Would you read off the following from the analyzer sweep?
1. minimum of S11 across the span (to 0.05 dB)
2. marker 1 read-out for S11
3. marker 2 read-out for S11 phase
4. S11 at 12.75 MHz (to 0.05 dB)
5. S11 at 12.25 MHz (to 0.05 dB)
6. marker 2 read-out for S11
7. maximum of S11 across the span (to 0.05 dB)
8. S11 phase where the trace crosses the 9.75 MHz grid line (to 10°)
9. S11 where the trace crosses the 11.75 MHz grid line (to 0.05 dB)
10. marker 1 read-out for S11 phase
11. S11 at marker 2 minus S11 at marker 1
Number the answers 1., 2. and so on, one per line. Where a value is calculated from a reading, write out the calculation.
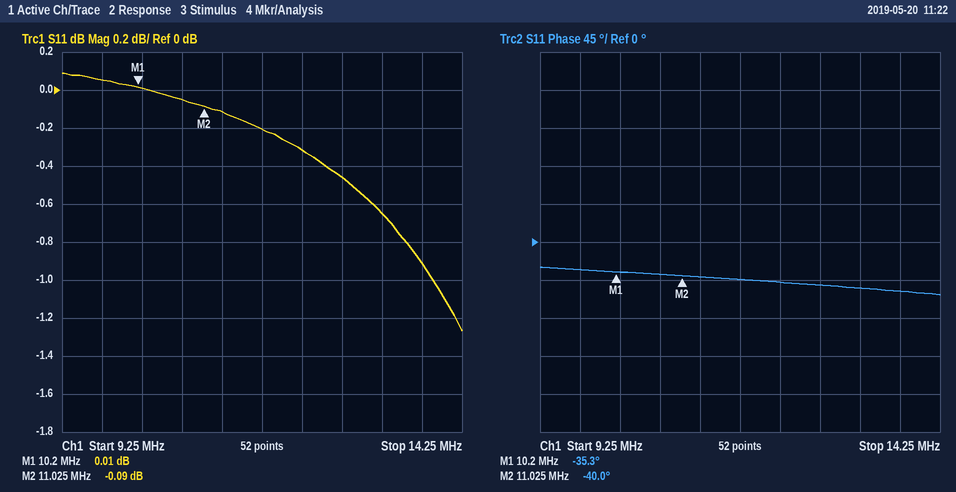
1. -1.25 dB
2. 0.01 dB
3. -40.0°
4. -0.45 dB
5. -0.30 dB
6. -0.09 dB
7. 0.10 dB
8. -30°
9. -0.20 dB
10. -35.3°
11. -0.09 − (0.01) = -0.10 dB
